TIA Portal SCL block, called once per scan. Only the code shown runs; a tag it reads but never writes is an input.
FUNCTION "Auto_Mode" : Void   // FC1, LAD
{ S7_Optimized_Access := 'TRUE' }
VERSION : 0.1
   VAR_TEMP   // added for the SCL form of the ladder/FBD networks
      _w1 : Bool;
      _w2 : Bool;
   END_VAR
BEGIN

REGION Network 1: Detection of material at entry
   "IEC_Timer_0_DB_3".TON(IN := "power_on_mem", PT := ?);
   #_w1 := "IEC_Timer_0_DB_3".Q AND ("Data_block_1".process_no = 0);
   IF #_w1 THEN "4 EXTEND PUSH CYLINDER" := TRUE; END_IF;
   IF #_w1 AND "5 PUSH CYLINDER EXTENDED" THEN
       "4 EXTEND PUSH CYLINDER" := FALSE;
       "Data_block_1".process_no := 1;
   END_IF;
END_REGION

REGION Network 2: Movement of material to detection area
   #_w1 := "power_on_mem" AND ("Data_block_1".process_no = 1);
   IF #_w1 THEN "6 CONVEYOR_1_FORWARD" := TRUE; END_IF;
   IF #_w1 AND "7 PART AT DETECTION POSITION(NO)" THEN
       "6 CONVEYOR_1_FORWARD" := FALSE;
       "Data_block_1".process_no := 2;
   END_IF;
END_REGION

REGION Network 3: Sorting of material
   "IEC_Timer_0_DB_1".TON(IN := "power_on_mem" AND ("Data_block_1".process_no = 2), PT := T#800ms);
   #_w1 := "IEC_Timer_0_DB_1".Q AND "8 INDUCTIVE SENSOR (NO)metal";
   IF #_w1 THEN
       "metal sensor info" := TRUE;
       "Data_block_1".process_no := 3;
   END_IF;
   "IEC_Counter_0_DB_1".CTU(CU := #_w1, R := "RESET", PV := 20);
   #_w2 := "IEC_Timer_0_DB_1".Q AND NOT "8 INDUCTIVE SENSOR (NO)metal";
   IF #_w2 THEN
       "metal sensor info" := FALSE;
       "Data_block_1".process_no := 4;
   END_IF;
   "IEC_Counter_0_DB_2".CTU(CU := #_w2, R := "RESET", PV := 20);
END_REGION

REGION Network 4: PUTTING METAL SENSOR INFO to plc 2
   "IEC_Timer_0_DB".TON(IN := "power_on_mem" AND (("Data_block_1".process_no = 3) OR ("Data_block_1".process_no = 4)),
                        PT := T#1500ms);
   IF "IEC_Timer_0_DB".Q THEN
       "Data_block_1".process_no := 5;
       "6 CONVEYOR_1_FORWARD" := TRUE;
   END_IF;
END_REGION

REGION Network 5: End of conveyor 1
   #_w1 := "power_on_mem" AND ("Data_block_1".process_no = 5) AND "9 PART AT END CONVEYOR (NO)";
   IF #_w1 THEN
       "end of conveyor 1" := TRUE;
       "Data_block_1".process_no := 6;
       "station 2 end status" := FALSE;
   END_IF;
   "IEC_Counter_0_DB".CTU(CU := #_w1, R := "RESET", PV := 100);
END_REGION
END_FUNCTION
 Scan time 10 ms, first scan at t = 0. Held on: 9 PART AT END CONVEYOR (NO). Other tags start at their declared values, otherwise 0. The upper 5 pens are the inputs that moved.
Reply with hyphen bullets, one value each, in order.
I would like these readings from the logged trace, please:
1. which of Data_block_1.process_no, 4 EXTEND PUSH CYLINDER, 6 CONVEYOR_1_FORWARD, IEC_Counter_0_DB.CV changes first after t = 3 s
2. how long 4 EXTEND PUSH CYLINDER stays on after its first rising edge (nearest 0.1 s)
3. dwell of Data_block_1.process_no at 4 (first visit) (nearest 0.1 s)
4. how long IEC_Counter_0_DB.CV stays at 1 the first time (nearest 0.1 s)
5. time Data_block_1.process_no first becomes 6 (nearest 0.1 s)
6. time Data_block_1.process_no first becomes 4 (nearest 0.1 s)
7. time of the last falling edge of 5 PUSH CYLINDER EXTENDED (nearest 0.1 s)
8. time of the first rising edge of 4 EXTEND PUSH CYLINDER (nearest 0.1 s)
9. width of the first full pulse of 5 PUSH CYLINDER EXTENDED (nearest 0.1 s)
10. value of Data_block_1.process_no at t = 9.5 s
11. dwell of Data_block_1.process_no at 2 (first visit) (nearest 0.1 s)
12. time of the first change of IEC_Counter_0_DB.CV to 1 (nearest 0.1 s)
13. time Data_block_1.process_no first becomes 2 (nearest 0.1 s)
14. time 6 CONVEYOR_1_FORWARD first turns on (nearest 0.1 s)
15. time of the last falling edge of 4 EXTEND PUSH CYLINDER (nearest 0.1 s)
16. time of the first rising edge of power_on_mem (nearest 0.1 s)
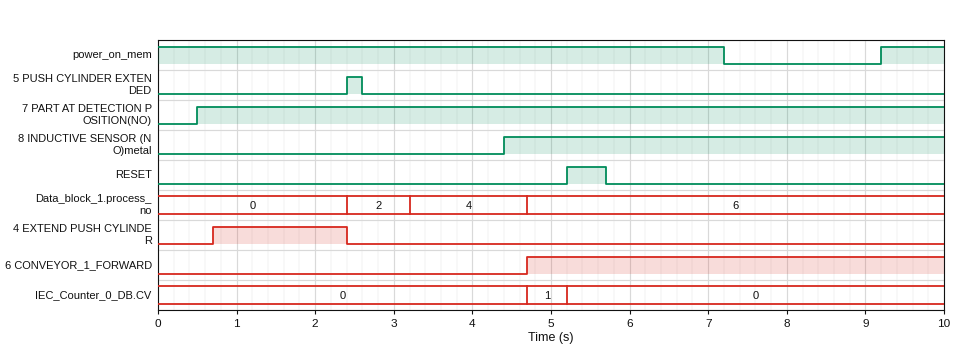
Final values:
- Data_block_1.process_no
- 1.7 s
- 1.5 s
- 0.5 s
- 4.7 s
- 3.2 s
- 2.6 s
- 0.7 s
- 0.2 s
- 6
- 0.8 s
- 4.7 s
- 2.4 s
- 4.7 s
- 2.4 s
- 9.2 s
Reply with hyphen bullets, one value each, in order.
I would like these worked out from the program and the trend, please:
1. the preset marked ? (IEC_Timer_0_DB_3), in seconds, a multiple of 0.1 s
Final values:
- 0.7 s
